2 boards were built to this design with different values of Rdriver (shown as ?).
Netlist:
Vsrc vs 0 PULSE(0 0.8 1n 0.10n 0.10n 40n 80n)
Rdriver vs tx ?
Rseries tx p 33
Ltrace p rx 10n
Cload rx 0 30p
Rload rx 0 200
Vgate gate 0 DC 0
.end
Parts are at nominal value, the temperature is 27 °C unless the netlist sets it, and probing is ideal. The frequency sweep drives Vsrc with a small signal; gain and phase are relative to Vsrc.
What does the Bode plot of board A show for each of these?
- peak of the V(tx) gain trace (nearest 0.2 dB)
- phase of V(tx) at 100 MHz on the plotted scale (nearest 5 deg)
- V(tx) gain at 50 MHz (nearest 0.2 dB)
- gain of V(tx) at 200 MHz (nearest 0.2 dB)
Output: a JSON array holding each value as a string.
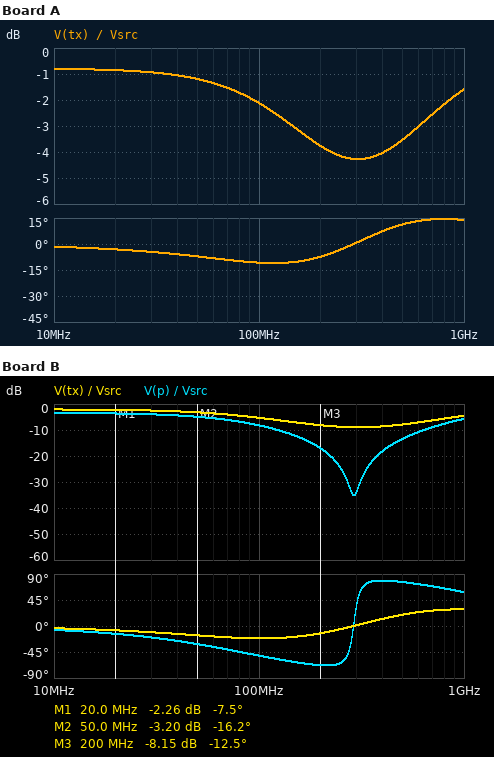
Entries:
["-0.8 dB", "-10 deg", "-1.2 dB", "-3.8 dB"]
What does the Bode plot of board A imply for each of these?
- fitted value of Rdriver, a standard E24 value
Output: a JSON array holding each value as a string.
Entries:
["22 Ω"]
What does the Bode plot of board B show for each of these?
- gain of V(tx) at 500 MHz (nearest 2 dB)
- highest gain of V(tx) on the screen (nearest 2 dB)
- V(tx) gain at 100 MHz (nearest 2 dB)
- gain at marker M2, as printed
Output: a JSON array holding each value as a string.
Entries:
["-8 dB", "-2 dB", "-6 dB", "-3.20 dB"]
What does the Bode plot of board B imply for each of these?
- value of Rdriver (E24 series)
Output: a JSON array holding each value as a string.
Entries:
["62 Ω"]
